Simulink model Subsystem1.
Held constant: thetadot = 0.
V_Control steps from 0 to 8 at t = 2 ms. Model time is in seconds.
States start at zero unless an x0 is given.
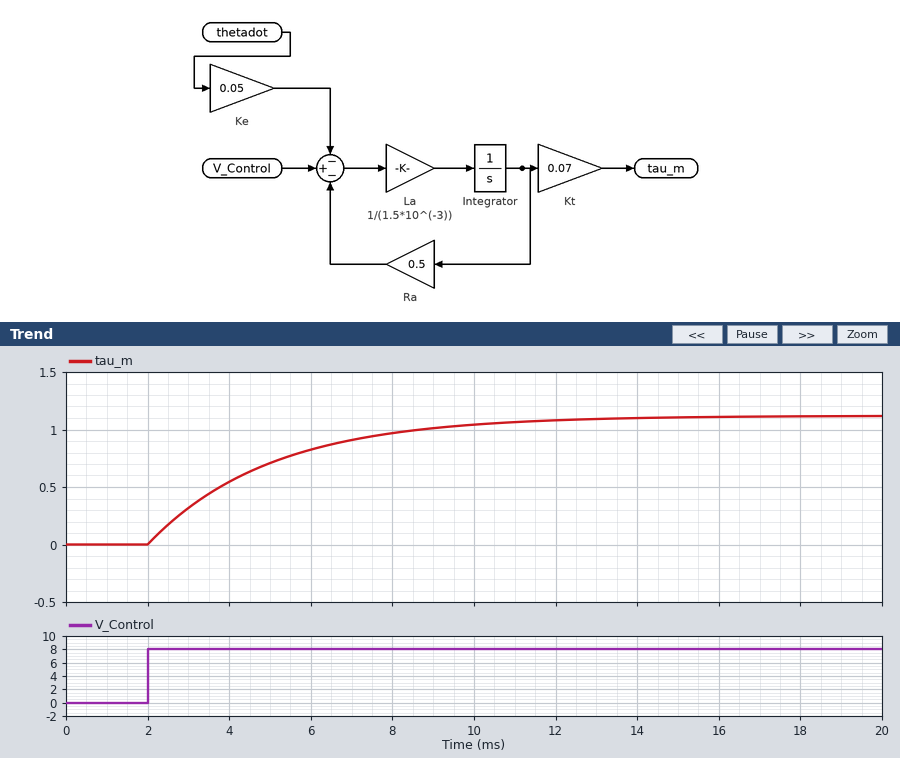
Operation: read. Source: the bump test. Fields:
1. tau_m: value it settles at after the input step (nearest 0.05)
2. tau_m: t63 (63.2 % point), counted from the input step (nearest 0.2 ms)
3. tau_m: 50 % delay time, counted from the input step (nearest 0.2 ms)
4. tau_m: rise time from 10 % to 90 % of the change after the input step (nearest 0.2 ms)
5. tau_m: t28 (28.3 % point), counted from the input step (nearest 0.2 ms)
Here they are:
1.10
3.0 ms
2.0 ms
6.6 ms
1.0 ms
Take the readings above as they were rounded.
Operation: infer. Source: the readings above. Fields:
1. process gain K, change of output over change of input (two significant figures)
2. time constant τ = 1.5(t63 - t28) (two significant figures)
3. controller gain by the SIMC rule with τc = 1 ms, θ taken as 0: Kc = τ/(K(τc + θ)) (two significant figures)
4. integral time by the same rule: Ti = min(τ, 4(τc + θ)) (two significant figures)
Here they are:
0.14
3.0 ms
21
3.0 ms
